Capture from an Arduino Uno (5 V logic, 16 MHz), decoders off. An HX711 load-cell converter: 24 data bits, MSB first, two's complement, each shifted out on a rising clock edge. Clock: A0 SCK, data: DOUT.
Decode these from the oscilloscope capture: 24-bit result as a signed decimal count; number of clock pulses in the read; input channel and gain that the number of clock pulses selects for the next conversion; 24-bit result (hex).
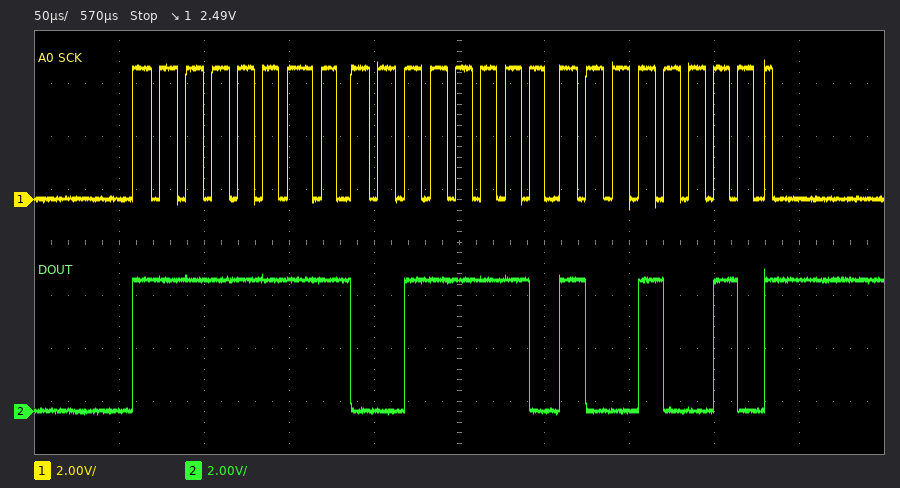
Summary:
-49518
25
channel A, gain 128
0xFF3E92
